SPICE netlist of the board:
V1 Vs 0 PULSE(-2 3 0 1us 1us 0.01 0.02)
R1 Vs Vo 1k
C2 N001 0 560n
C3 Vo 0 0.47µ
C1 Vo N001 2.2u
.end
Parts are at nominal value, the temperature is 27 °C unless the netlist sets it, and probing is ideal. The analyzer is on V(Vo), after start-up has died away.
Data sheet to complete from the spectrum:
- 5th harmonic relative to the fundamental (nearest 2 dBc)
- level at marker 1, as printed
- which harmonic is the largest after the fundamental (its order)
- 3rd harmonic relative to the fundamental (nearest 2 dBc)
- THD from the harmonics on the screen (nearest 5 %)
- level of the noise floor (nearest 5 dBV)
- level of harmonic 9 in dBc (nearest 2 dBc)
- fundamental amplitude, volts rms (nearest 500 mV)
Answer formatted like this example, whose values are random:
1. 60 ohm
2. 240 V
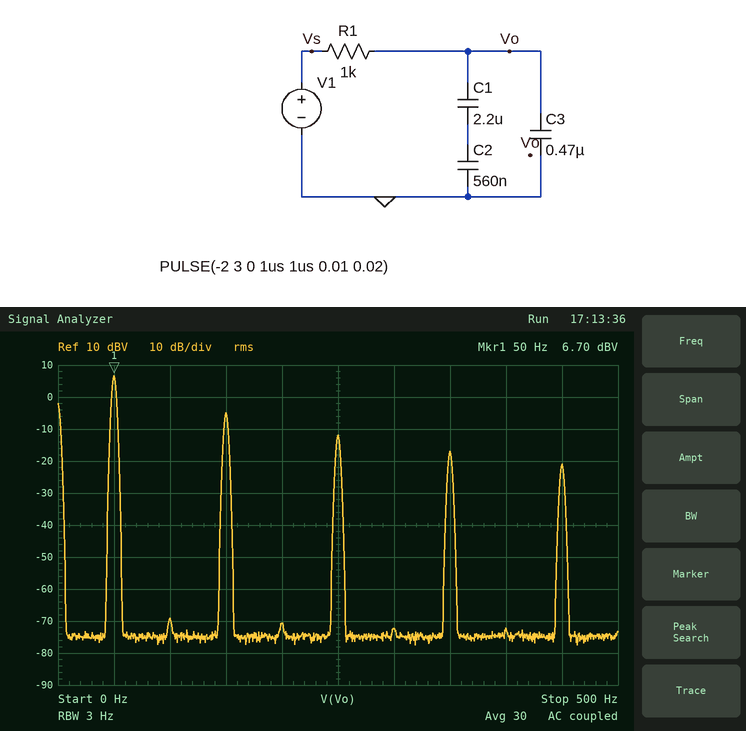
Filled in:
1. -18 dBc
2. 6.70 dBV
3. 3
4. -12 dBc
5. 30 %
6. -75 dBV
7. -28 dBc
8. 2.0 V
